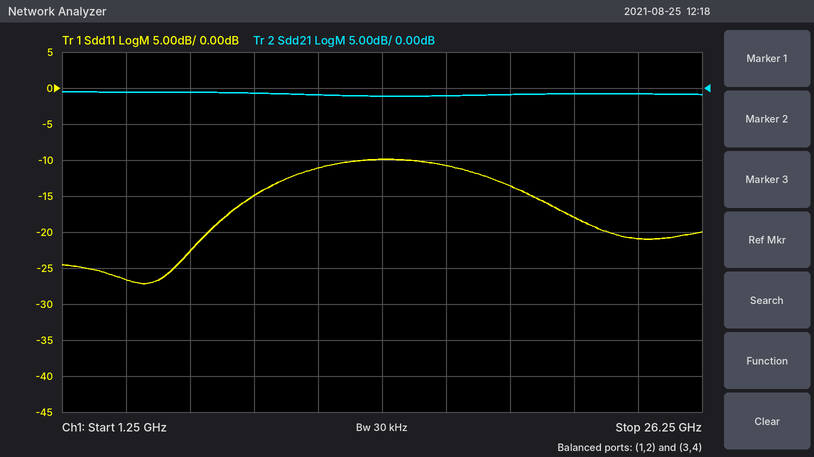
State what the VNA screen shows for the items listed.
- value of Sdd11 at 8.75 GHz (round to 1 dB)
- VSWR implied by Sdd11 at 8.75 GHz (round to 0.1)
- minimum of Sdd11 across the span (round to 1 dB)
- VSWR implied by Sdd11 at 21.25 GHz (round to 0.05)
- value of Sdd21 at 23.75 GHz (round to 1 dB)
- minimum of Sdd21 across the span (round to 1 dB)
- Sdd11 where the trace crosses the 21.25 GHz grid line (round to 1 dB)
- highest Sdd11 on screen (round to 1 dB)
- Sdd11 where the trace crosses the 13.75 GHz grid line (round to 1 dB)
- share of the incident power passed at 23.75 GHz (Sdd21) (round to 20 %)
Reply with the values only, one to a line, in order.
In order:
-15 dB
1.4
-27 dB
1.30
-1 dB
-1 dB
-18 dB
-10 dB
-10 dB
80 %
